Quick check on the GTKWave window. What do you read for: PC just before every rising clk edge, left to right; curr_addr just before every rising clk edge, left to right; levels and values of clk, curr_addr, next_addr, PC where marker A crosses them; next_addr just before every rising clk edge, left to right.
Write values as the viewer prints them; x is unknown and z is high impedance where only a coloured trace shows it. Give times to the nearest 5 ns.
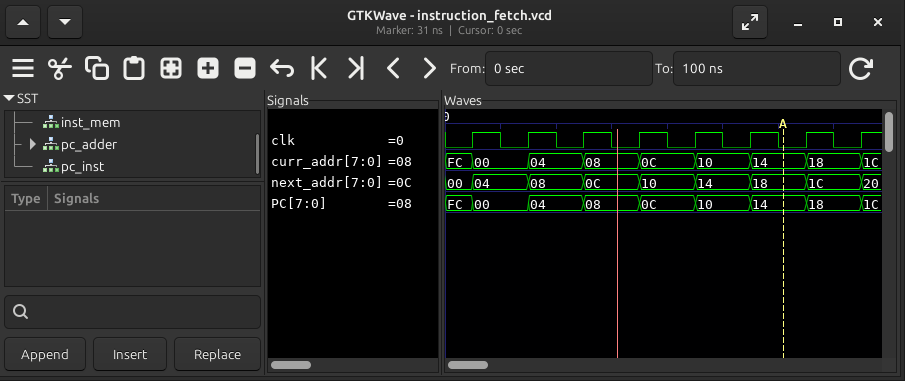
FC, 00, 04, 08, 0C, 10, 14, 18
FC, 00, 04, 08, 0C, 10, 14, 18
clk=0, curr_addr=14, next_addr=18, PC=14
00, 04, 08, 0C, 10, 14, 18, 1C
